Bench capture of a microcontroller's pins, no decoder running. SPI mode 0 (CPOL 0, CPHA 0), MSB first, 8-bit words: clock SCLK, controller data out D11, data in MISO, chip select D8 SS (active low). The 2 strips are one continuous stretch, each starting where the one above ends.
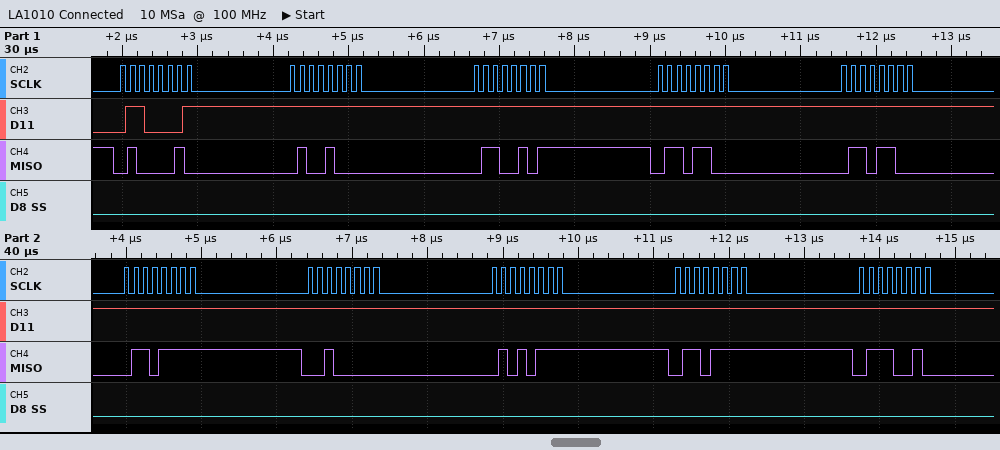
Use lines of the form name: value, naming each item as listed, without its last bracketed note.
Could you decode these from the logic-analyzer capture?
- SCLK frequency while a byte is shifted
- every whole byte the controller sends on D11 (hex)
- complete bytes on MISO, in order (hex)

SCLK frequency while a byte is shifted: 8 MHz
every whole byte the controller sends on D11: 61 FF FF FF FF FF FF FF FF FF
complete bytes on MISO, in order: 42 48 65 6C 6C 6F 20 57 6F 72
